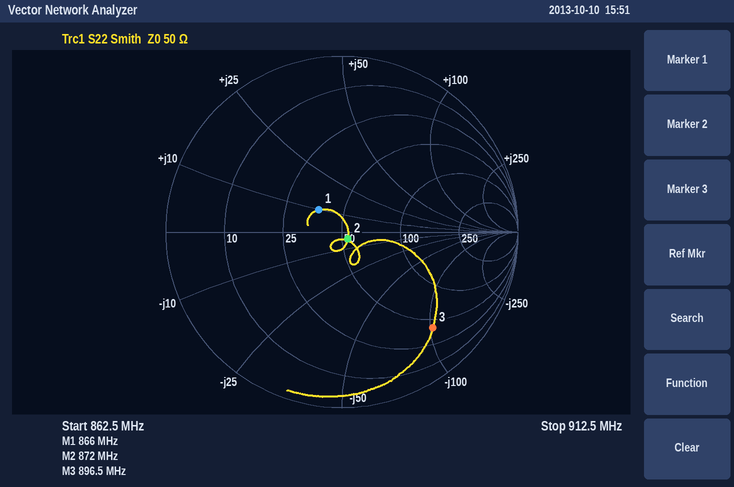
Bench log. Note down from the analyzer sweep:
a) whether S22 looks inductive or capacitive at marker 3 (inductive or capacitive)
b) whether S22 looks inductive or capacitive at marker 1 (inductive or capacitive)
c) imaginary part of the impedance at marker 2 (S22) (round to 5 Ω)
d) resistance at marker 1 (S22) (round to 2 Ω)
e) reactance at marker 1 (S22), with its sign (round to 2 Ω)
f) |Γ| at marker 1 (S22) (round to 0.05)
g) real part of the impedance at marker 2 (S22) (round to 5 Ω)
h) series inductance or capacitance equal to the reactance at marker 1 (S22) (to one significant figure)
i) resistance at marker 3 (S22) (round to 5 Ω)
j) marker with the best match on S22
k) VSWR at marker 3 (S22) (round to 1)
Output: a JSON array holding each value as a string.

["capacitive", "inductive", "-5 Ω", "38 Ω", "+10 Ω", "0.20", "55 Ω", "2 nH", "40 Ω", "marker 2", "7"]
